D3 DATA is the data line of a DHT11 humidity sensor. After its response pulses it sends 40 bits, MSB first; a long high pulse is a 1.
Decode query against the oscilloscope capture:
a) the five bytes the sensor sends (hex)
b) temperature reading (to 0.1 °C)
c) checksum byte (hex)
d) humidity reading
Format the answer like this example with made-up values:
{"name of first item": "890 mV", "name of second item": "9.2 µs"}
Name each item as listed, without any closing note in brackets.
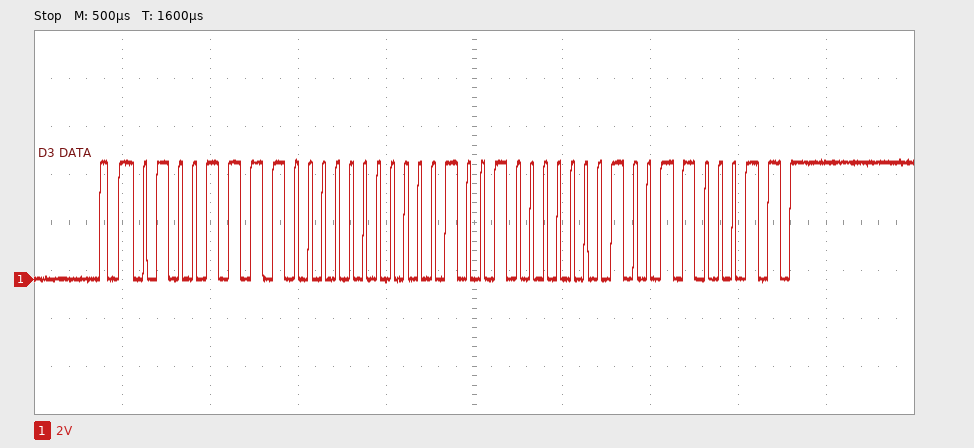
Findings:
{"the five bytes the sensor sends": "4F 00 12 02 63", "temperature reading": "18.2 °C", "checksum byte": "0x63", "humidity reading": "79 %"}
